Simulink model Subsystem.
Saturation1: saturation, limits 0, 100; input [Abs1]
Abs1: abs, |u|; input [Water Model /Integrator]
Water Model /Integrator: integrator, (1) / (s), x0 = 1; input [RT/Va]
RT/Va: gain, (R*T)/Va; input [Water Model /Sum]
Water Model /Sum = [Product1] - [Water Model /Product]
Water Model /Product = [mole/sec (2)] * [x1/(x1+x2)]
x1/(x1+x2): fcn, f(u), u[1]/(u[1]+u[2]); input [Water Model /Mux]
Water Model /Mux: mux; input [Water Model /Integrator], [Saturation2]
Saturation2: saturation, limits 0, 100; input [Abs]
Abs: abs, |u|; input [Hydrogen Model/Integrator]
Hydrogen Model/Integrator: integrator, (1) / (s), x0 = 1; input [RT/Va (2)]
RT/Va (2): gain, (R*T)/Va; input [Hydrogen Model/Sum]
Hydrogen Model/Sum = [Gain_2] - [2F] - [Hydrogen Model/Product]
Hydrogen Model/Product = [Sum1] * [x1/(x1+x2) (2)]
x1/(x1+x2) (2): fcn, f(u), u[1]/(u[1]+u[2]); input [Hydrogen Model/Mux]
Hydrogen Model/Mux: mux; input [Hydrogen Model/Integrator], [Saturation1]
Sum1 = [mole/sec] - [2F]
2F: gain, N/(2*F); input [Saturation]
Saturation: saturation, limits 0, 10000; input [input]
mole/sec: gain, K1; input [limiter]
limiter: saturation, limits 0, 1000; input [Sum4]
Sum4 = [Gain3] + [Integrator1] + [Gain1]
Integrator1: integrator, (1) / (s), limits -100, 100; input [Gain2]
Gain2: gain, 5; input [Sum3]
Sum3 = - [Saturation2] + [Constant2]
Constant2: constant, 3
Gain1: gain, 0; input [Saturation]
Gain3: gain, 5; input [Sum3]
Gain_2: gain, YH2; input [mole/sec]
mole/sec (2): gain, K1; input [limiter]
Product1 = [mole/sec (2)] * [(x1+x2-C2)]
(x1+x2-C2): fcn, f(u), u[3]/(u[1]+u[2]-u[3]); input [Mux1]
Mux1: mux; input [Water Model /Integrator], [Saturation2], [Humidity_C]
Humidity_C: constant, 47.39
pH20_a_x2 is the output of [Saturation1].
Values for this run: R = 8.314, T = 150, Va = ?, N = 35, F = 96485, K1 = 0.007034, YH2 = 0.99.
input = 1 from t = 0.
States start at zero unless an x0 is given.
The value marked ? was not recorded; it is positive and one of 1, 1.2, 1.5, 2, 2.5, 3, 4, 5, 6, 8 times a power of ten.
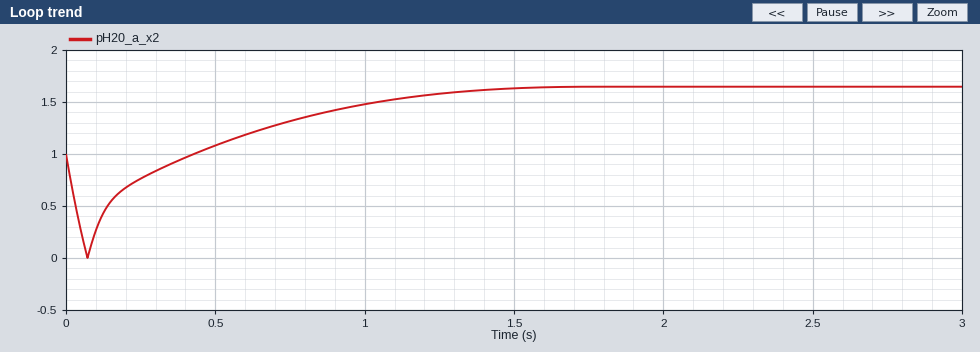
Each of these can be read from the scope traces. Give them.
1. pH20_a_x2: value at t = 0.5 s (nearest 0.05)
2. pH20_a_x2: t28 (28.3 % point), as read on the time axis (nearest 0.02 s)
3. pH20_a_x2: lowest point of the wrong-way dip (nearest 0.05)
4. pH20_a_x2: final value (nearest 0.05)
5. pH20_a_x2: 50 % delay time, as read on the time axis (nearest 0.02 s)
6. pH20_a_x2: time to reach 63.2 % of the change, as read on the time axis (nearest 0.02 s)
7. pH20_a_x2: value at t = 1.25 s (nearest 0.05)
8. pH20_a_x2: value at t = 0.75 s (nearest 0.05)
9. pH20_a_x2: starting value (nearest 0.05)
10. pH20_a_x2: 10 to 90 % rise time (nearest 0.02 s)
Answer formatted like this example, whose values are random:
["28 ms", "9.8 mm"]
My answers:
["1.10", "0.60 s", "0.00", "1.65", "0.76 s", "0.88 s", "1.60", "1.30", "1.00", "0.78 s"]
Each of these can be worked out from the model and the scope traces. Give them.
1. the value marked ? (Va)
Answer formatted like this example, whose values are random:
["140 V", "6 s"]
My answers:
["8"]
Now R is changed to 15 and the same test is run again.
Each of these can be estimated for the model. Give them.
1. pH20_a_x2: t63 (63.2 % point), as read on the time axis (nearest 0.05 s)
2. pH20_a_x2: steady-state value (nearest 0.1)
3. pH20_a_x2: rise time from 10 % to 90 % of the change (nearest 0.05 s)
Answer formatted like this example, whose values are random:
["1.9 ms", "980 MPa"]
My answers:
["0.55 s", "1.6", "0.50 s"]
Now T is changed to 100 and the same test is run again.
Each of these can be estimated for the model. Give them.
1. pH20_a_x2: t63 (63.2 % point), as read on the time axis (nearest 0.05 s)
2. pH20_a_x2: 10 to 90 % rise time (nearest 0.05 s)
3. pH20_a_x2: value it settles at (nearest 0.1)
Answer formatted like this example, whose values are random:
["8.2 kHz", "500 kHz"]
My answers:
["1.20 s", "1.00 s", "1.7"]
